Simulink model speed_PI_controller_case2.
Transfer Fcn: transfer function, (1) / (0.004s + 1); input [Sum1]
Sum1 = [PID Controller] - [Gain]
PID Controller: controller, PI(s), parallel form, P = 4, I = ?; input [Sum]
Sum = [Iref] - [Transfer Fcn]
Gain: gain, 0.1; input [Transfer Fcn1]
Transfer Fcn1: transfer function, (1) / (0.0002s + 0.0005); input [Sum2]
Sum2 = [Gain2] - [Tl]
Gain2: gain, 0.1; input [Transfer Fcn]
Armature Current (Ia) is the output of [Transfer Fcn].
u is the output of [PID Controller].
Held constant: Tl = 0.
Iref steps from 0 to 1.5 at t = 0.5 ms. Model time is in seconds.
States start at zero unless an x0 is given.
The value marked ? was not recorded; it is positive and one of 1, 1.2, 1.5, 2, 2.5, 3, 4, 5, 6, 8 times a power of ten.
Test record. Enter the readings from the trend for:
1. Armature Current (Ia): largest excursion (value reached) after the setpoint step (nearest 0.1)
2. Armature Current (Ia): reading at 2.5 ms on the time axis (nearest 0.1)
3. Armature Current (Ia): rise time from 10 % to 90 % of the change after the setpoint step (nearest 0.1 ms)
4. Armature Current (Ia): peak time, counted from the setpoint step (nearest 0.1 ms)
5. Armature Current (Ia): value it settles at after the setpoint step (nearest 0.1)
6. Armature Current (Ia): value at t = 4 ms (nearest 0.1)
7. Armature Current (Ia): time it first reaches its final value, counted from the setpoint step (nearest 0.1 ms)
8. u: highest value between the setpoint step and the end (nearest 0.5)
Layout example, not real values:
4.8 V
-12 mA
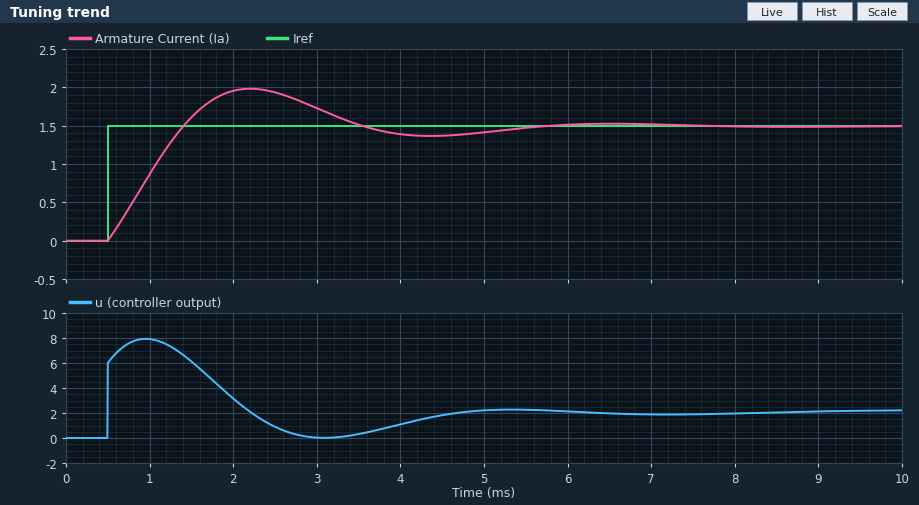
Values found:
2.0
1.9
0.7 ms
1.7 ms
1.5
1.4
0.9 ms
8.0
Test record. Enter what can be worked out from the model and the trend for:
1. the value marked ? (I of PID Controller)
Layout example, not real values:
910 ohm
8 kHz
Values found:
10000
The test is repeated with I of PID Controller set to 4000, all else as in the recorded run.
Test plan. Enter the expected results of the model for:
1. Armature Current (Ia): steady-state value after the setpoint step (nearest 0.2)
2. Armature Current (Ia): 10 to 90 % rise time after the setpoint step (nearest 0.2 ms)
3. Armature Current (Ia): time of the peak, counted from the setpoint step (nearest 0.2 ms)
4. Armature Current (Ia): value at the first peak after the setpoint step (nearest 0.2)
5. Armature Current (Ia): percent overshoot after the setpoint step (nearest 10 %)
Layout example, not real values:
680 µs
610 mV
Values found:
1.4
1.0 ms
2.6 ms
1.8
20 %
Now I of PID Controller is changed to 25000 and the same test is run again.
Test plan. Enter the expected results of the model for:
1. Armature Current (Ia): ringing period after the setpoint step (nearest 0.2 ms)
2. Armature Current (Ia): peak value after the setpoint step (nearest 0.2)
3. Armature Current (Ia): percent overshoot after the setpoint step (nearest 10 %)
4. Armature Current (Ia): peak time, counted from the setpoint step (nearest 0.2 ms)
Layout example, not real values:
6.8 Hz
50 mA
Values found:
2.6 ms
2.2
50 %
1.2 ms
